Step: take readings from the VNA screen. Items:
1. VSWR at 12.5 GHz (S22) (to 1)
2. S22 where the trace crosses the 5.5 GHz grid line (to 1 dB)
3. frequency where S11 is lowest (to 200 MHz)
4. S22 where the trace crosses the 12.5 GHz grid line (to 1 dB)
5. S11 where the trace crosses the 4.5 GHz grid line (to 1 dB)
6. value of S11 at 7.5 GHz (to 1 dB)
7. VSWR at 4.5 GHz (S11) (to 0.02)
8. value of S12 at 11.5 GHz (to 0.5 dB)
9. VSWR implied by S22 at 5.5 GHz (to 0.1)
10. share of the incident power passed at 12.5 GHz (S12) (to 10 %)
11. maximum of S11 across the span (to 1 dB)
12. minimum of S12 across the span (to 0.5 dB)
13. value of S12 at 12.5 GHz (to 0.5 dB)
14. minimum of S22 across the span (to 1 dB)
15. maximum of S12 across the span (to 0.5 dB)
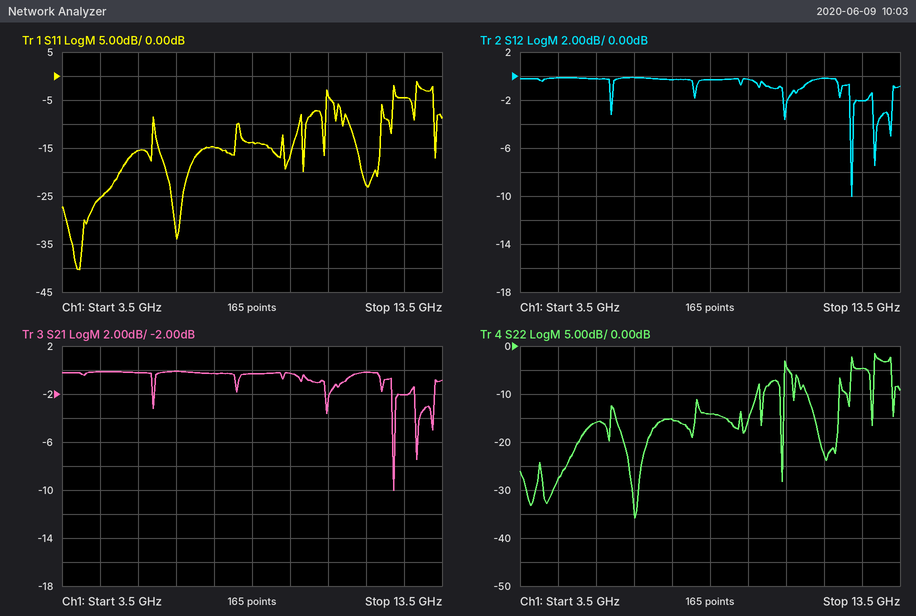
4
-16 dB
4.0 GHz
-5 dB
-25 dB
-15 dB
1.12
0.0 dB
1.4
60 %
-1 dB
-10.0 dB
-2.0 dB
-36 dB
0.0 dB
